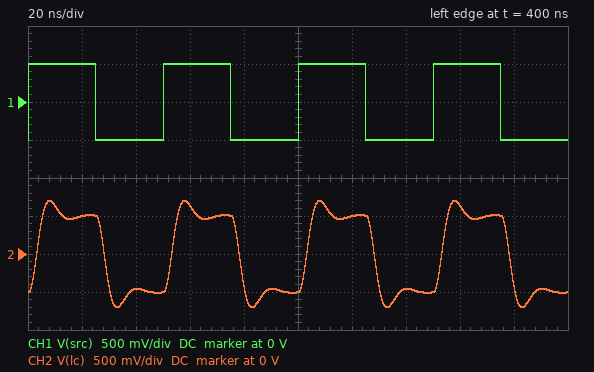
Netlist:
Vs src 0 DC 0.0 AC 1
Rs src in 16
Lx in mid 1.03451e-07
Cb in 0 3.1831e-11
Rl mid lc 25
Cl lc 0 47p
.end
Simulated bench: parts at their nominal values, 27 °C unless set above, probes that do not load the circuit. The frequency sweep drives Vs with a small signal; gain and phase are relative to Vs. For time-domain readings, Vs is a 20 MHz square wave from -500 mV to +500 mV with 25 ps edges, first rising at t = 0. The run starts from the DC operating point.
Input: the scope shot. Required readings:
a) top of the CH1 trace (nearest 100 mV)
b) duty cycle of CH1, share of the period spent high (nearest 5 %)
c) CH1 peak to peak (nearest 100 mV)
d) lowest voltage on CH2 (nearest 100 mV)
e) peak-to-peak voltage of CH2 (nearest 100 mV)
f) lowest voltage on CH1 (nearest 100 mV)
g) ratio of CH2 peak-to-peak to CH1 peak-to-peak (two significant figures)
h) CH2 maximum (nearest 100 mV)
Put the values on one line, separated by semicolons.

500 mV; 50 %; 1.0 V; -700 mV; 1.4 V; -500 mV; 1.4; 700 mV
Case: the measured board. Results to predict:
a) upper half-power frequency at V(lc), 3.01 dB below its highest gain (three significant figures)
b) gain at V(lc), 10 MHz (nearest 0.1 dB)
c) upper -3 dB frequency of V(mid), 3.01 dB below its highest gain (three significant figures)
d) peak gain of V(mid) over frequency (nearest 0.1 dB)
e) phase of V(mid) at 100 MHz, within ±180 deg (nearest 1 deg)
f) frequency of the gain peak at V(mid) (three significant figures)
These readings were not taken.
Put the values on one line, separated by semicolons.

88.4 MHz; 0.1 dB; 93.5 MHz; 2.5 dB; -105 deg; 61.7 MHz
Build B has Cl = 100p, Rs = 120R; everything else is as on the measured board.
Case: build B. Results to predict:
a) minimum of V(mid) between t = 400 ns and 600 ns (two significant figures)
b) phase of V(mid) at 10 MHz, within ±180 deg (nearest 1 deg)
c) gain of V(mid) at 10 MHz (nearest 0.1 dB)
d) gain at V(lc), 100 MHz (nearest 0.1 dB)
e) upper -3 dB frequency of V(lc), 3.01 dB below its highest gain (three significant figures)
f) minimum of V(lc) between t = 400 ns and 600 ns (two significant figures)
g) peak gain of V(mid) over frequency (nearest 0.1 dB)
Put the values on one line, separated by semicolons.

-330 mV; -42 deg; -3.2 dB; -17.0 dB; 9.31 MHz; -310 mV; 0 dB
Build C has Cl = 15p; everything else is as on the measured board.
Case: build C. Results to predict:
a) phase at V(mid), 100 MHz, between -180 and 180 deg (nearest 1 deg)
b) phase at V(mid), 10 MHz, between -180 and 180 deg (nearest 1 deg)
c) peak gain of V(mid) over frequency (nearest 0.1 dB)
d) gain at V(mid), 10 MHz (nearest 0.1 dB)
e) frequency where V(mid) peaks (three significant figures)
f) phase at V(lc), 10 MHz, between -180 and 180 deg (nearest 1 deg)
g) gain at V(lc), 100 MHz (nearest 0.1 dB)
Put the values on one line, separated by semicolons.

-45 deg; -3 deg; 6.3 dB; 0 dB; 125 MHz; -4 deg; 4.5 dB
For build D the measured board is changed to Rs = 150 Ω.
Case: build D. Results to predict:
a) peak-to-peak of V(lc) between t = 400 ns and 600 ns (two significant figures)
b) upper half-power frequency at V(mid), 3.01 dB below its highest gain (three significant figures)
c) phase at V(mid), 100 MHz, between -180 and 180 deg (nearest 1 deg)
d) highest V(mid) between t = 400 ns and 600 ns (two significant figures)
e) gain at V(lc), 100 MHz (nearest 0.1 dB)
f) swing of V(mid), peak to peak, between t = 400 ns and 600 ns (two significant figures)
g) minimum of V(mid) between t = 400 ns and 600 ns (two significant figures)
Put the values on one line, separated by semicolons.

770 mV; 13.4 MHz; -106 deg; 390 mV; -11.9 dB; 780 mV; -390 mV
